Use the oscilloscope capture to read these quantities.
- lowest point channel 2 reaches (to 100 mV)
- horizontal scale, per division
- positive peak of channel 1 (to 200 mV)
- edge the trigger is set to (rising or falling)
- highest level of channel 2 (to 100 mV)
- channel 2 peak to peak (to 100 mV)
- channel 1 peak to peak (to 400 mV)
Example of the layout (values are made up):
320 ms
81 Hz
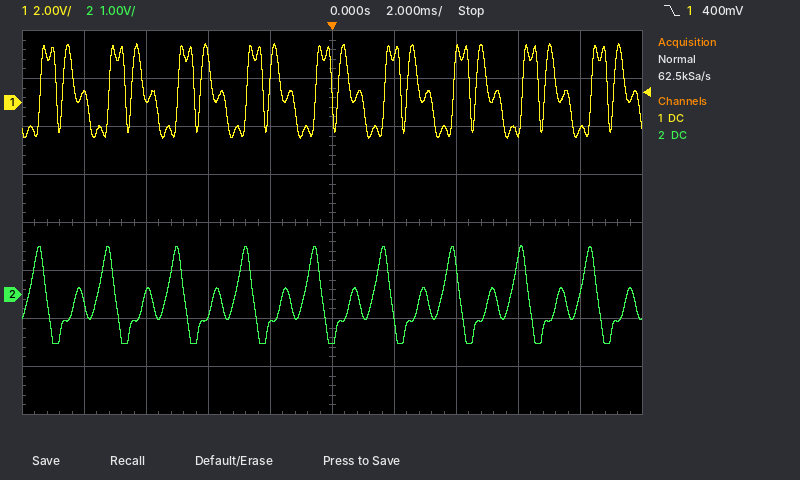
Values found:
-1.0 V
2 ms
2.4 V
falling
1.0 V
2.0 V
4.0 V
